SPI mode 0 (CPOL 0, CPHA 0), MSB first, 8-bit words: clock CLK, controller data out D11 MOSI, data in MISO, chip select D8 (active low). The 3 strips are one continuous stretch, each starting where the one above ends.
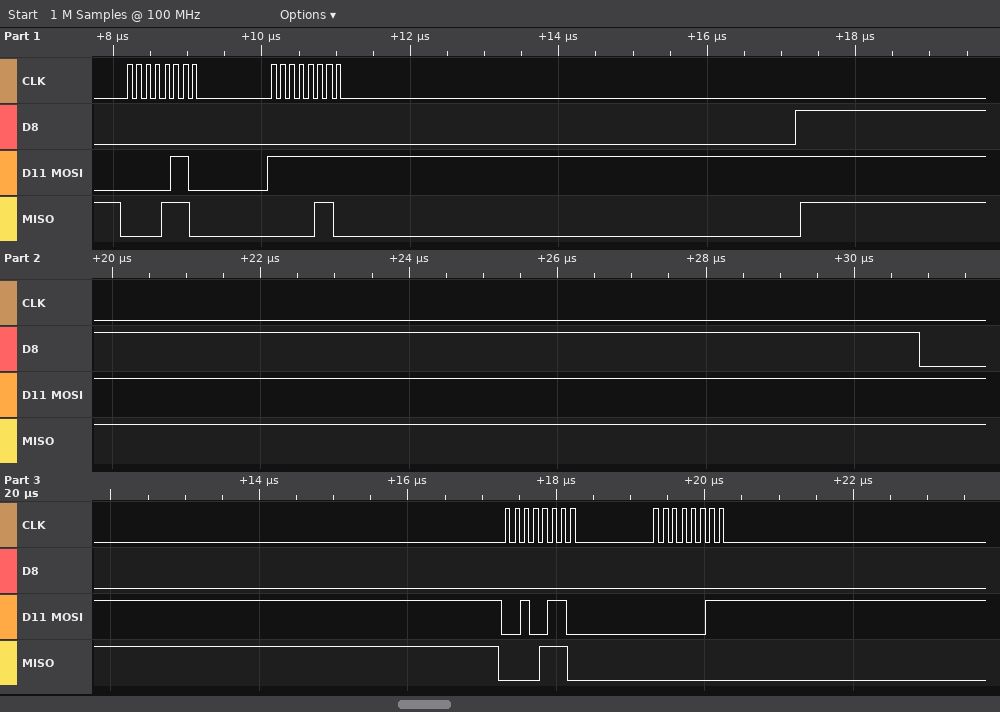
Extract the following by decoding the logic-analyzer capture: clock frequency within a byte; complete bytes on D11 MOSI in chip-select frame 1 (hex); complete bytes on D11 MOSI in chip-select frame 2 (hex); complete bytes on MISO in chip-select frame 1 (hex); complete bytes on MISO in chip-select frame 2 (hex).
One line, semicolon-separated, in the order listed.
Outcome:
8 MHz; 0x06 0xFF; 0x26 0x03; 0x0E 0x06; 0x0E 0x00
